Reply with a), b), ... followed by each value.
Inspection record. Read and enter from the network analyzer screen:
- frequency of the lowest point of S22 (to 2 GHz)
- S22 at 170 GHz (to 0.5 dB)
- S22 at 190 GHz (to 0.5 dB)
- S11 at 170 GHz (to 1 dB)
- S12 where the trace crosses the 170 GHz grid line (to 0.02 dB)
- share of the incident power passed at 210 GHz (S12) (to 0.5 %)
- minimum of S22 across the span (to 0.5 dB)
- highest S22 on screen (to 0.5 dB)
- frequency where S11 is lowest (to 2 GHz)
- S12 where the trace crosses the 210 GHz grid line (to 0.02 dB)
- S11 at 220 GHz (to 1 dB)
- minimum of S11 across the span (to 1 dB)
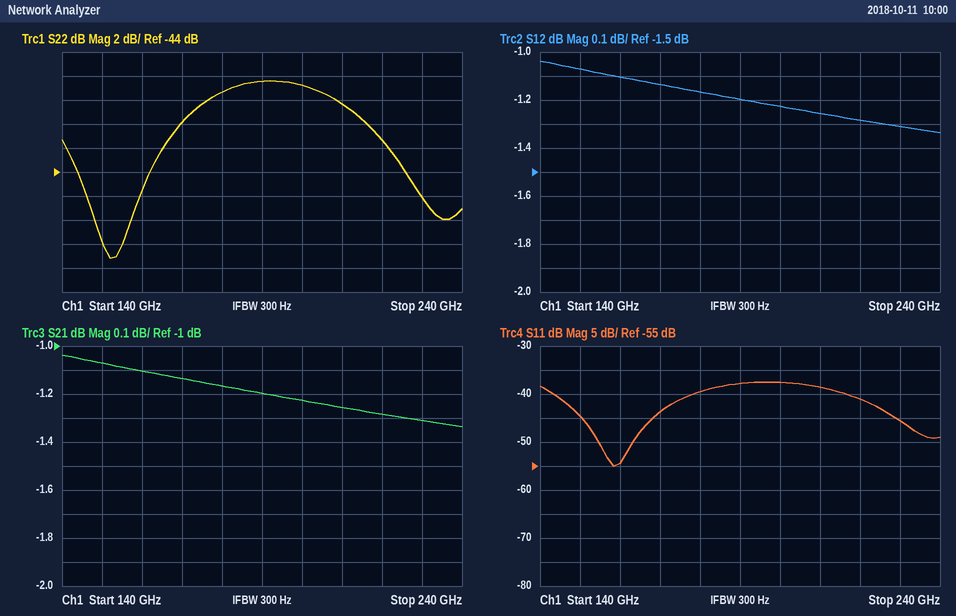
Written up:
a) 152 GHz
b) -40.0 dB
c) -36.5 dB
d) -44 dB
e) -1.14 dB
f) 75.0 %
g) -51.0 dB
h) -36.5 dB
i) 158 GHz
j) -1.26 dB
k) -41 dB
l) -55 dB
